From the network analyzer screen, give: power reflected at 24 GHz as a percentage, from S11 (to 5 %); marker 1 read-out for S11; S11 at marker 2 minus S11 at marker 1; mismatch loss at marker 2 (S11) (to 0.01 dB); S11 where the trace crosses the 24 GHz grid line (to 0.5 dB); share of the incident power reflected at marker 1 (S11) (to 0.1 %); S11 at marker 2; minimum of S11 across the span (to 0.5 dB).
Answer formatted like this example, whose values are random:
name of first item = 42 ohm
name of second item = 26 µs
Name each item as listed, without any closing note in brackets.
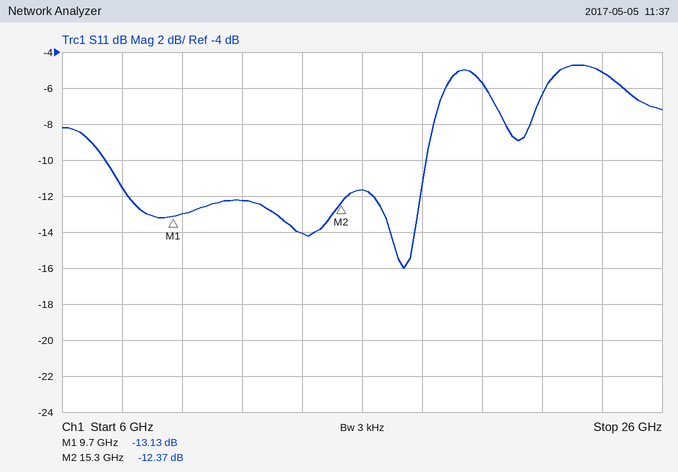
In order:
power reflected at 24 GHz as a percentage, from S11 = 30 %
marker 1 read-out for S11 = -13.13 dB
S11 at marker 2 minus S11 at marker 1 = 0.76 dB
mismatch loss at marker 2 (S11) = 0.26 dB
S11 where the trace crosses the 24 GHz grid line = -5.0 dB
share of the incident power reflected at marker 1 (S11) = 4.9 %
S11 at marker 2 = -12.37 dB
minimum of S11 across the span = -16.0 dB
